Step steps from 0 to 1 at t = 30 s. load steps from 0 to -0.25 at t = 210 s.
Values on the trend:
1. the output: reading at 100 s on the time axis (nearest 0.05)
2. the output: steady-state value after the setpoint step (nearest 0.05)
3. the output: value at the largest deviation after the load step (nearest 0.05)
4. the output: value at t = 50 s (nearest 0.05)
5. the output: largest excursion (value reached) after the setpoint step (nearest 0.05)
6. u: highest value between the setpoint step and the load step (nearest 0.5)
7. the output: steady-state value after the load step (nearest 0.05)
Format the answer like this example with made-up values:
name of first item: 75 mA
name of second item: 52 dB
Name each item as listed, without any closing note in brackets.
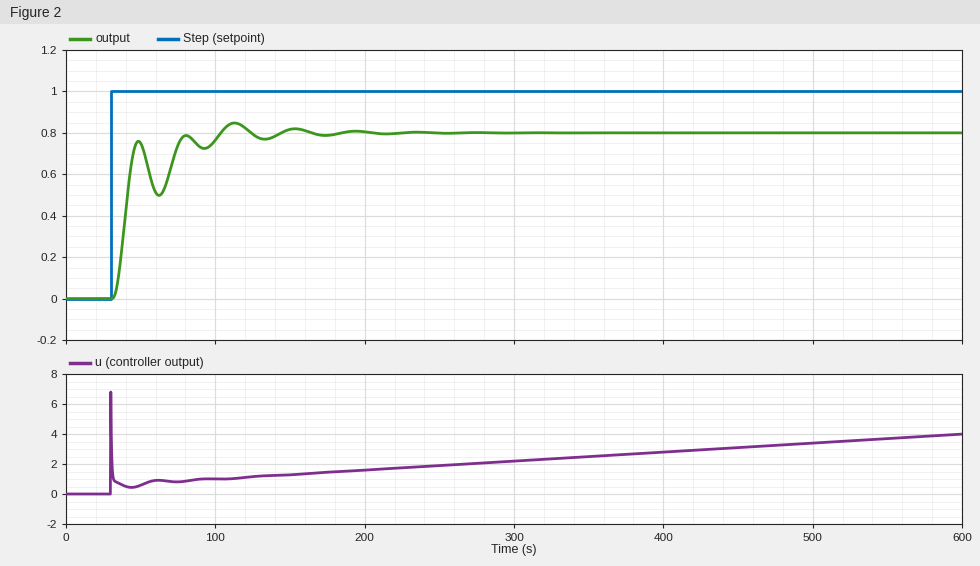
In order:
the output: reading at 100 s on the time axis: 0.75
the output: steady-state value after the setpoint step: 0.80
the output: value at the largest deviation after the load step: 0.80
the output: value at t = 50 s: 0.75
the output: largest excursion (value reached) after the setpoint step: 0.85
u: highest value between the setpoint step and the load step: 7.0
the output: steady-state value after the load step: 0.80
